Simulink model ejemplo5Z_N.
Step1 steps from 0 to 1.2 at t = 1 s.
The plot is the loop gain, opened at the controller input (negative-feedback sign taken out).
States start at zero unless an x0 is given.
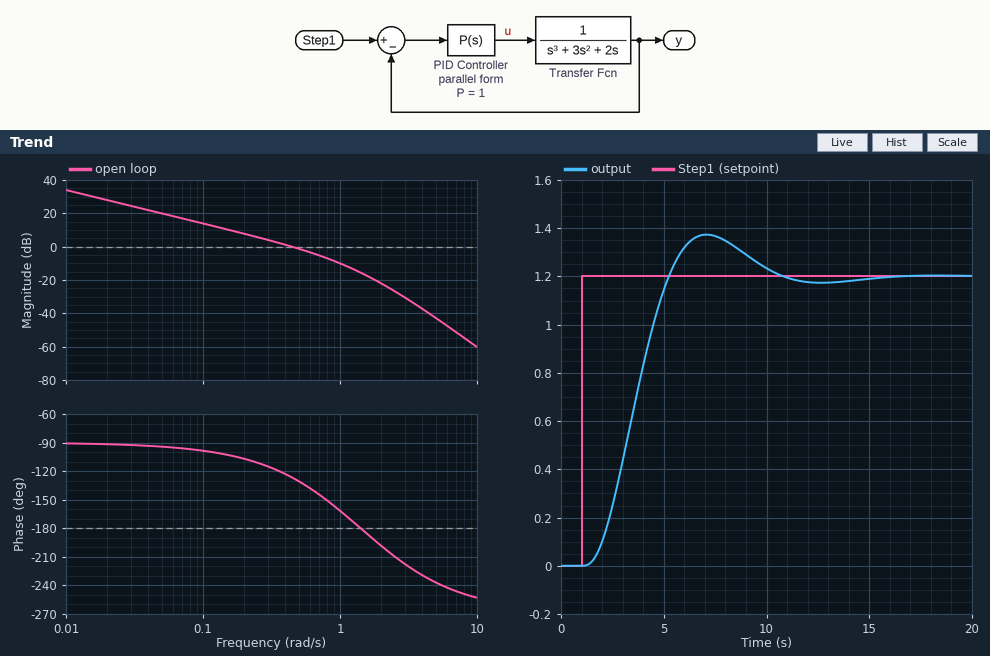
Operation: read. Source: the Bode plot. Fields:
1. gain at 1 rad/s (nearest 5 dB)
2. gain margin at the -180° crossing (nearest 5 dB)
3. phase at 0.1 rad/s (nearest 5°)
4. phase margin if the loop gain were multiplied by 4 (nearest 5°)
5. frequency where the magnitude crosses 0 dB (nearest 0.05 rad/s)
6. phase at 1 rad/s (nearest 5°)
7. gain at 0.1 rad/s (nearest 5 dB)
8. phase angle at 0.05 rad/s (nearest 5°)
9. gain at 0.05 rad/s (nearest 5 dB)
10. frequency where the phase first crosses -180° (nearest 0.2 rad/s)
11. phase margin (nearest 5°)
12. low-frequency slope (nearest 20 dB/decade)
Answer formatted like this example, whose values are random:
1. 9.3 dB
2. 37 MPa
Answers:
1. -10 dB
2. 15 dB
3. -100°
4. 10°
5. 0.45 rad/s
6. -160°
7. 15 dB
8. -95°
9. 20 dB
10. 1.4 rad/s
11. 55°
12. -20 dB/decade
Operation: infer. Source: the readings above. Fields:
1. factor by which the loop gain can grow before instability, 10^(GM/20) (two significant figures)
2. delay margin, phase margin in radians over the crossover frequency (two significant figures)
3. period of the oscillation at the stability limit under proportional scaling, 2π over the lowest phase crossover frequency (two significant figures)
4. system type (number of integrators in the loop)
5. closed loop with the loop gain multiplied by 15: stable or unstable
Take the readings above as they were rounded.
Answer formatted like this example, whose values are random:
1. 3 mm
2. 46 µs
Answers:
1. 5.6
2. 2.1 s
3. 4.5 s
4. 1
5. unstable
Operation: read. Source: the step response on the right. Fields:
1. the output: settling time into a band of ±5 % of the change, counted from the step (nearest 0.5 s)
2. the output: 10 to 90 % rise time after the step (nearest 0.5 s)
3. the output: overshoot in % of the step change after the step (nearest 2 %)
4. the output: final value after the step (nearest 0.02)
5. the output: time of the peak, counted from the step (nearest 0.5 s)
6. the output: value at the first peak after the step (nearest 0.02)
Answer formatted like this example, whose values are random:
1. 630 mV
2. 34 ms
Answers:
1. 8.5 s
2. 2.5 s
3. 14 %
4. 1.20
5. 6.0 s
6. 1.38
